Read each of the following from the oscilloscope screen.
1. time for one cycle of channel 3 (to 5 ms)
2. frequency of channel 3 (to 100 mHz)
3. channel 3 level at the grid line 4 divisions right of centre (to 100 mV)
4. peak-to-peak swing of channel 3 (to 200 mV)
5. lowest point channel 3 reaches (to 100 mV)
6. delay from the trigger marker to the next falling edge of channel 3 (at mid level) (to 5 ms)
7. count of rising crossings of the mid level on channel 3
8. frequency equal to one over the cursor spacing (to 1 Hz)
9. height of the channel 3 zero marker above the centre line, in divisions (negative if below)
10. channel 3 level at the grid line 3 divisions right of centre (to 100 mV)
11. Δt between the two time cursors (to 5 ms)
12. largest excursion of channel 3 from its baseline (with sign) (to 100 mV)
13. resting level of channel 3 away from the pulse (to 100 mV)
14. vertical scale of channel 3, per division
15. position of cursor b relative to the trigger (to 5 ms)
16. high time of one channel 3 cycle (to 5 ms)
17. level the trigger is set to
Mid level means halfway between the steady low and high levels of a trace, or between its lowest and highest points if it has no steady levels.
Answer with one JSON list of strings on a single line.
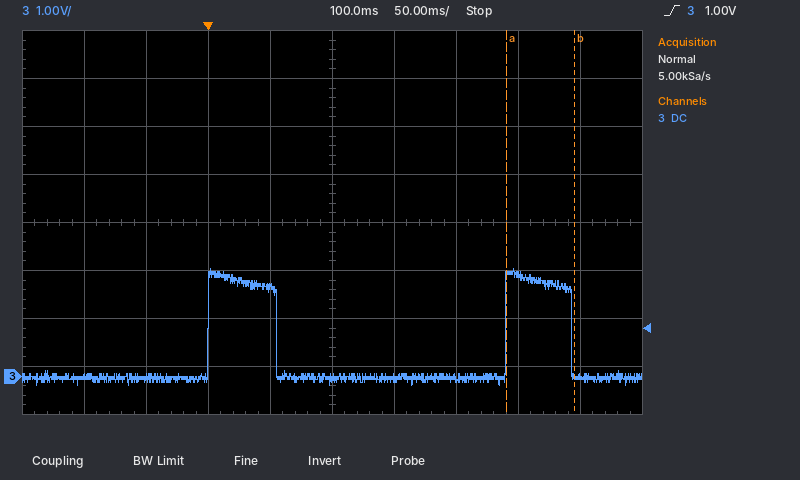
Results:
["240 ms", "4.2 Hz", "0.0 V", "2.4 V", "-200 mV", "55 ms", "2", "18 Hz", "-3.2 div", "2.1 V", "55 ms", "+2.3 V", "0.0 V", "1 V", "+295 ms", "55 ms", "1.00 V"]
